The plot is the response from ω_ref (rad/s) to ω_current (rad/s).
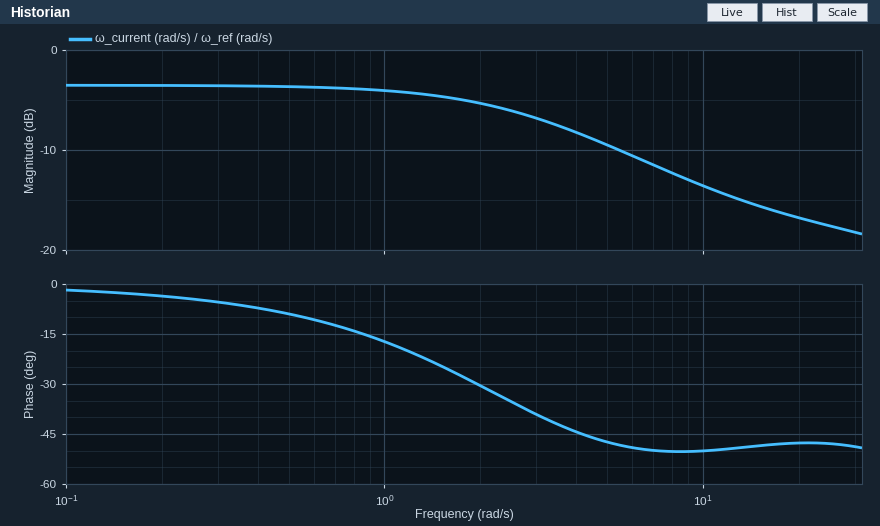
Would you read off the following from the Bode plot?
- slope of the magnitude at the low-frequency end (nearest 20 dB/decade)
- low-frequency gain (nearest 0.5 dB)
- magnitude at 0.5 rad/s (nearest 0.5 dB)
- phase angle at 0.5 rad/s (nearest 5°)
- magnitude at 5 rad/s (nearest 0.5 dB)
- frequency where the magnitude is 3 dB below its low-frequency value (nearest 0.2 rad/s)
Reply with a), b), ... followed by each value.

a) 0 dB/decade
b) -3.5 dB
c) -3.5 dB
d) -10°
e) -9.5 dB
f) 2.8 rad/s
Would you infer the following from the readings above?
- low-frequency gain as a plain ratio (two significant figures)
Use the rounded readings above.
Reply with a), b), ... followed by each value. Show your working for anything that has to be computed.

a) 10^(-3.5 / 20) = 0.67
